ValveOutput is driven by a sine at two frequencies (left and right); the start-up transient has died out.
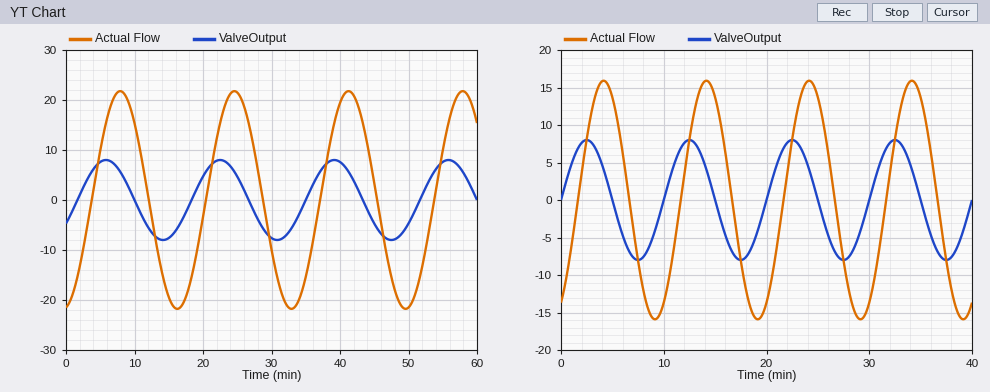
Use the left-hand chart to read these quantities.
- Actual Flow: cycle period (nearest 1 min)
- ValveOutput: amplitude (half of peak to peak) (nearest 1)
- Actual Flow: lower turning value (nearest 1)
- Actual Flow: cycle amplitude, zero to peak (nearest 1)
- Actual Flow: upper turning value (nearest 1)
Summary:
17 min
8
-22
22
22
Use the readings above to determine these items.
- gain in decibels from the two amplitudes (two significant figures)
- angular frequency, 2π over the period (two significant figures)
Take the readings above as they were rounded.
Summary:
8.8 dB
0.37 rad/min
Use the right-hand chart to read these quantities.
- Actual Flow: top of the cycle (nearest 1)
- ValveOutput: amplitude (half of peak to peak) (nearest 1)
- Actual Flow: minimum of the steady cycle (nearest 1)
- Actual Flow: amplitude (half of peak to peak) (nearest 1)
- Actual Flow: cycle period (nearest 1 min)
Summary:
16
8
-16
16
10 min
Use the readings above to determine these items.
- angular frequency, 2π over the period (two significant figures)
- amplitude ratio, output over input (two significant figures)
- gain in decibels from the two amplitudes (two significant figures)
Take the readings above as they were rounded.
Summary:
0.63 rad/min
2.0
6.0 dB
